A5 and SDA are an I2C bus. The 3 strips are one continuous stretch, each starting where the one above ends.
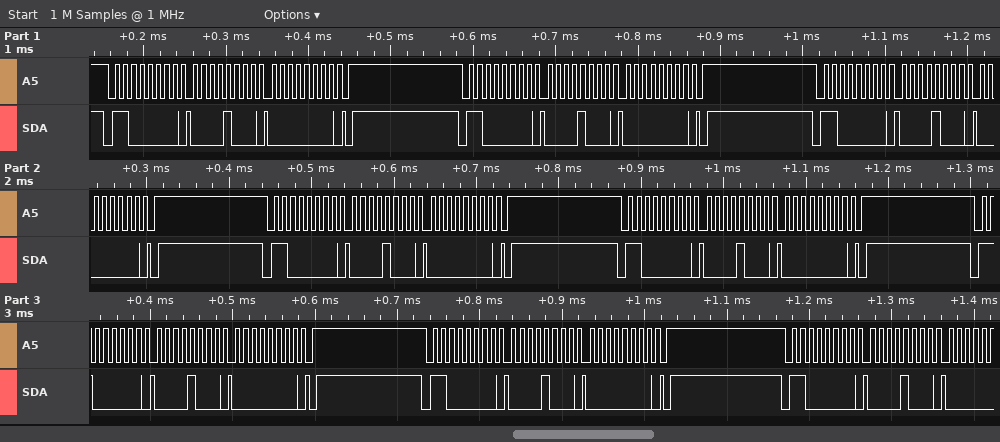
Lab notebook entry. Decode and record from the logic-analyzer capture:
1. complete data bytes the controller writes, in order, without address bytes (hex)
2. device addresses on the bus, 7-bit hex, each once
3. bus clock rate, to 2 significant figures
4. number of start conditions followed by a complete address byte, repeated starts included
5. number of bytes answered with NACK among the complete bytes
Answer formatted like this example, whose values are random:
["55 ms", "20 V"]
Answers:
["08 00 08 00 08 00 08 00 08 00 08 00 08 00 08", "0x60", "100 kHz", "8", "0"]
